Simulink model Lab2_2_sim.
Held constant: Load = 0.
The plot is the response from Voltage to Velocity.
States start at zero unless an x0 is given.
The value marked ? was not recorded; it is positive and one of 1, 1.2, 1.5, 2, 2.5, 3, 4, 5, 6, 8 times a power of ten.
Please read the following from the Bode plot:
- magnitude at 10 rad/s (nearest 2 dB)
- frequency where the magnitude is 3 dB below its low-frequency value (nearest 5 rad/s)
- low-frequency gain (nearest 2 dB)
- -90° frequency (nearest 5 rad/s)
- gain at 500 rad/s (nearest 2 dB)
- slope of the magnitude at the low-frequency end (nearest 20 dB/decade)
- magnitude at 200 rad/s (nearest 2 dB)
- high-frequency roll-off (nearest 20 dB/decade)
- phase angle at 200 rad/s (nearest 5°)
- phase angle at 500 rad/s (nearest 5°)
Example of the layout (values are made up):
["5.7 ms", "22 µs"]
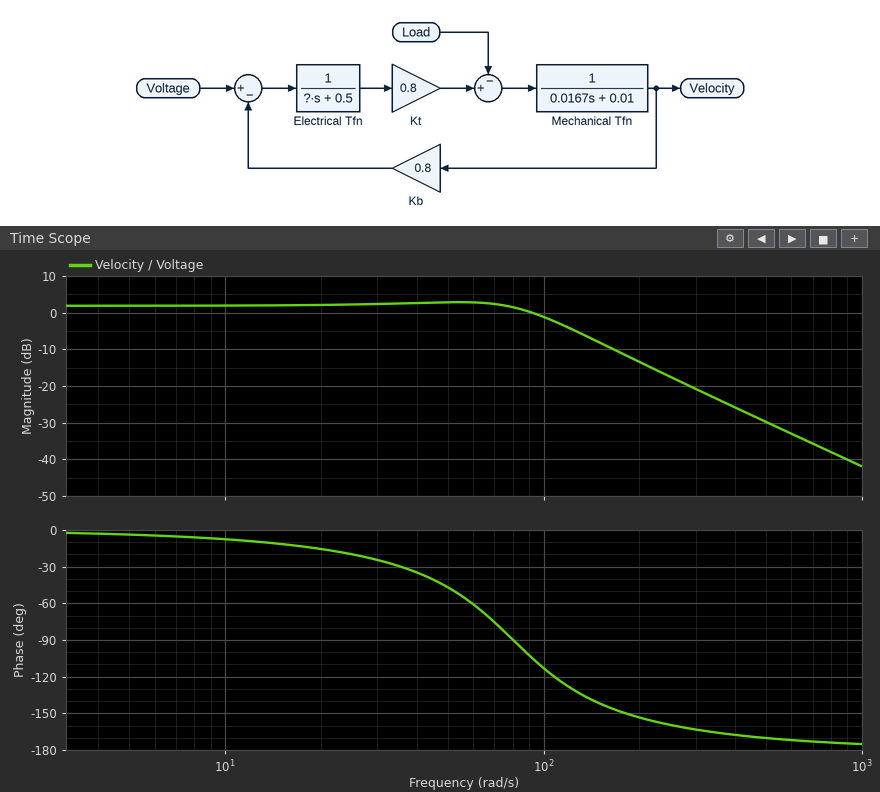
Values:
["2 dB", "100 rad/s", "2 dB", "80 rad/s", "-30 dB", "0 dB/decade", "-14 dB", "-40 dB/decade", "-155°", "-170°"]
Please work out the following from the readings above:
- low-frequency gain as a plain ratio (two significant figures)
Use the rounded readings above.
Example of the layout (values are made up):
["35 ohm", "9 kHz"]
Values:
["1.3"]
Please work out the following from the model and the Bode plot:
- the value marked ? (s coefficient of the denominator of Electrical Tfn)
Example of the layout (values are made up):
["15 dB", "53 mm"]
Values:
["0.006"]
